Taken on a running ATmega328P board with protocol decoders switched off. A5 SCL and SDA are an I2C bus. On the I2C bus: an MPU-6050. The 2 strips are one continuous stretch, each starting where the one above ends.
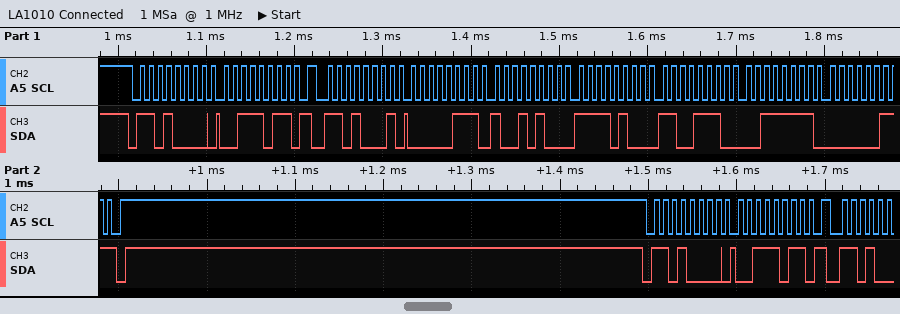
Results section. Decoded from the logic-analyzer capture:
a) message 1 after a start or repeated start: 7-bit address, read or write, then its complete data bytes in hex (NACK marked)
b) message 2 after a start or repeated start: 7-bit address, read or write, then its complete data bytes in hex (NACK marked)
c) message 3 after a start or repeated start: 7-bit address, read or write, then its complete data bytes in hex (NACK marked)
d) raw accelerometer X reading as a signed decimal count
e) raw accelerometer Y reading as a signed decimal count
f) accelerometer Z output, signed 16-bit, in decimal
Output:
0x68 write: 3B
0x68 read: 07 94 F4 CE 3F 03 NACK
0x68 write: 3B
1940
-2866
16131
